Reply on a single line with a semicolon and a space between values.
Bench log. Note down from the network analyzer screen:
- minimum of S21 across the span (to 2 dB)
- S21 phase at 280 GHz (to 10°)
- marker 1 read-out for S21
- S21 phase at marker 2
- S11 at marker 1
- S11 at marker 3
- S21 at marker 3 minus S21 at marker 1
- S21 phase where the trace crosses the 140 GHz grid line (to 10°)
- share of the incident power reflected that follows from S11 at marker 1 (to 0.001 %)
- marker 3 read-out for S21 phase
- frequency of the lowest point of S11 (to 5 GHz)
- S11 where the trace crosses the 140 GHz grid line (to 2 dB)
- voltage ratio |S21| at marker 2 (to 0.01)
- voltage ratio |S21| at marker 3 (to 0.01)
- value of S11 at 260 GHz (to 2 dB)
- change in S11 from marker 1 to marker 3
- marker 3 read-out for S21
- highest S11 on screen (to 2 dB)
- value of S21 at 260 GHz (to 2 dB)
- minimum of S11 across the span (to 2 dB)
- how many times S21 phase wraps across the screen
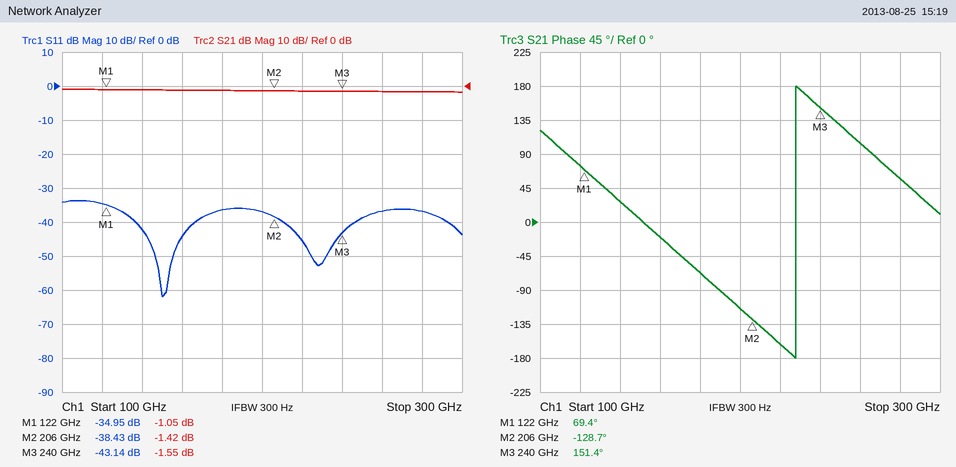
-2 dB; 60°; -1.05 dB; -128.7°; -34.95 dB; -43.14 dB; -0.50 dB; 30°; 0.032 %; 151.4°; 150 GHz; -42 dB; 0.85; 0.84; -36 dB; -8.19 dB; -1.55 dB; -34 dB; -2 dB; -62 dB; 1
